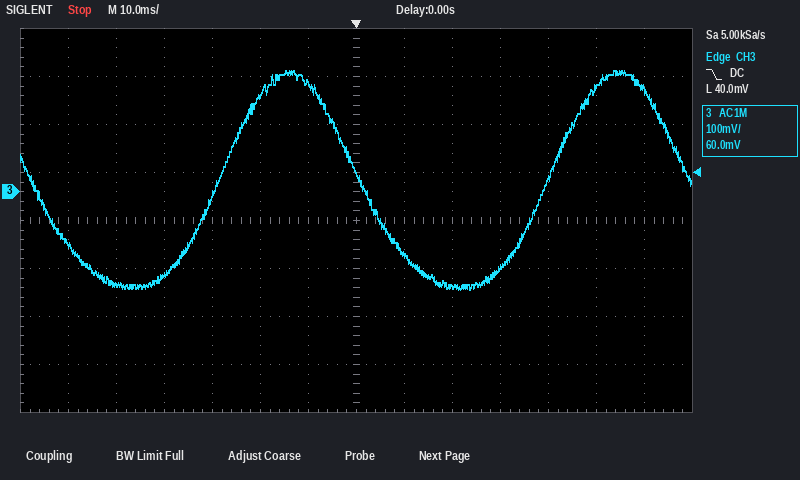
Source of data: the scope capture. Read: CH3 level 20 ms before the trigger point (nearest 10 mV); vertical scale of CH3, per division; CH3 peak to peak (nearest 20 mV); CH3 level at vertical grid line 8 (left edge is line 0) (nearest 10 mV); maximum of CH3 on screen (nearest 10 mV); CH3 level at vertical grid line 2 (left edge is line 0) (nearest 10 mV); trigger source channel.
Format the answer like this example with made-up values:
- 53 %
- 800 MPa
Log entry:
- 200 mV
- 100 mV
- 460 mV
- -130 mV
- 250 mV
- -190 mV
- CH3
